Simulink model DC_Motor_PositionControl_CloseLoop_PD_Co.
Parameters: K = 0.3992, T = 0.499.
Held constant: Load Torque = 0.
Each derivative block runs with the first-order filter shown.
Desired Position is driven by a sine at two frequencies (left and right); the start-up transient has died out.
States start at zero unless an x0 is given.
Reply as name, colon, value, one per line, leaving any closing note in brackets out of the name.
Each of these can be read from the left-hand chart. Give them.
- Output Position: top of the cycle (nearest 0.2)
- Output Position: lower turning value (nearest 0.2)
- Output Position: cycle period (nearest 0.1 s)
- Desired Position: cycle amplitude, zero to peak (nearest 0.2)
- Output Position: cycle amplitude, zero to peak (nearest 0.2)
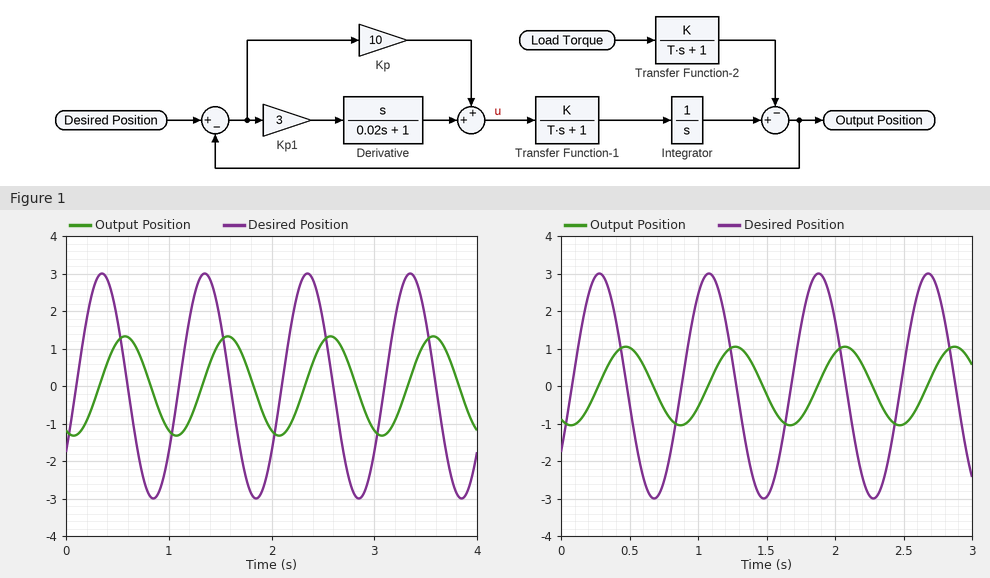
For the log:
Output Position: top of the cycle: 1.4
Output Position: lower turning value: -1.4
Output Position: cycle period: 1.0 s
Desired Position: cycle amplitude, zero to peak: 3.0
Output Position: cycle amplitude, zero to peak: 1.4
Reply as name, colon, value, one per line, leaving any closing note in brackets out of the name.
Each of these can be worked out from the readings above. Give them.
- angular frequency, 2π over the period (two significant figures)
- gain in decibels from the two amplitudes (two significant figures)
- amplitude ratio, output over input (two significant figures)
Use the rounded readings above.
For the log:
angular frequency, 2π over the period: 6.3 rad/s
gain in decibels from the two amplitudes: -6.6 dB
amplitude ratio, output over input: 0.47
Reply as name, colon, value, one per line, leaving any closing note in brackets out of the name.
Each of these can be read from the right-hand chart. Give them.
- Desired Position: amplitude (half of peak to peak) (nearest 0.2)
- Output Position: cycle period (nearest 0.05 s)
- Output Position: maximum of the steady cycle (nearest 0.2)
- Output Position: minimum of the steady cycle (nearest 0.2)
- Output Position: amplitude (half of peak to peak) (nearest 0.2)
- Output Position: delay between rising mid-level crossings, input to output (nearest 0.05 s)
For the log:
Desired Position: amplitude (half of peak to peak): 3.0
Output Position: cycle period: 0.80 s
Output Position: maximum of the steady cycle: 1.0
Output Position: minimum of the steady cycle: -1.0
Output Position: amplitude (half of peak to peak): 1.0
Output Position: delay between rising mid-level crossings, input to output: 0.20 s
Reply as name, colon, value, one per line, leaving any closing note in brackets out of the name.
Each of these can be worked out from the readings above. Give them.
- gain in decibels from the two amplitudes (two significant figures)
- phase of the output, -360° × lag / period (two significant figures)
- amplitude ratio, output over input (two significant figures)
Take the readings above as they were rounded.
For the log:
gain in decibels from the two amplitudes: -9.5 dB
phase of the output, -360° × lag / period: -90°
amplitude ratio, output over input: 0.33
